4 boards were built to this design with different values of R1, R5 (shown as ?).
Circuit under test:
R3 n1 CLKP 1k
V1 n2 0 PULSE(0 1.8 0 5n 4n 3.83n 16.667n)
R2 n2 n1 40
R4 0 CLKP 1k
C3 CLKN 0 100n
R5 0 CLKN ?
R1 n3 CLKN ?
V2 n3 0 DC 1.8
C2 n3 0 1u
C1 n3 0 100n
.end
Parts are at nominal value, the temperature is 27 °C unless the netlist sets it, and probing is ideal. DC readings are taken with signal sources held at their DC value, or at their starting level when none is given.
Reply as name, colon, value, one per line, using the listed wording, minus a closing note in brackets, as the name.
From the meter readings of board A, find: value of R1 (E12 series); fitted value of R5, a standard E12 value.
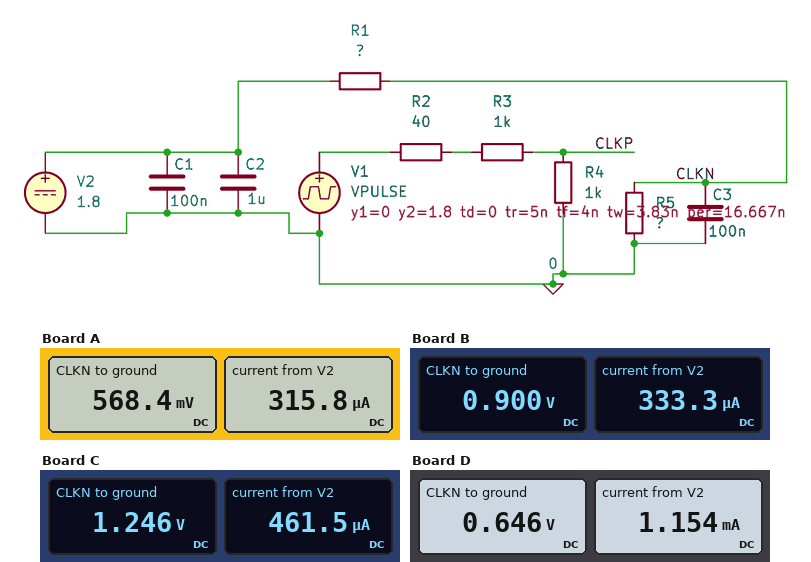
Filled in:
value of R1: 3.9 kΩ
fitted value of R5, a standard E12 value: 1.8 kΩ
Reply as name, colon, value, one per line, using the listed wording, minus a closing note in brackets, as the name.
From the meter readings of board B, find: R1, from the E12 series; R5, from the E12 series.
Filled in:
R1, from the E12 series: 2.7 kΩ
R5, from the E12 series: 2.7 kΩ
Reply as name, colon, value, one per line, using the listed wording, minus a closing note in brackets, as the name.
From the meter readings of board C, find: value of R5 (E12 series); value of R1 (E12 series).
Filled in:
value of R5: 2.7 kΩ
value of R1: 1.2 kΩ
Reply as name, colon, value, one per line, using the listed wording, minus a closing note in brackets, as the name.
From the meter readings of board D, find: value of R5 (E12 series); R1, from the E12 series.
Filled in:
value of R5: 560 Ω
R1, from the E12 series: 1 kΩ
